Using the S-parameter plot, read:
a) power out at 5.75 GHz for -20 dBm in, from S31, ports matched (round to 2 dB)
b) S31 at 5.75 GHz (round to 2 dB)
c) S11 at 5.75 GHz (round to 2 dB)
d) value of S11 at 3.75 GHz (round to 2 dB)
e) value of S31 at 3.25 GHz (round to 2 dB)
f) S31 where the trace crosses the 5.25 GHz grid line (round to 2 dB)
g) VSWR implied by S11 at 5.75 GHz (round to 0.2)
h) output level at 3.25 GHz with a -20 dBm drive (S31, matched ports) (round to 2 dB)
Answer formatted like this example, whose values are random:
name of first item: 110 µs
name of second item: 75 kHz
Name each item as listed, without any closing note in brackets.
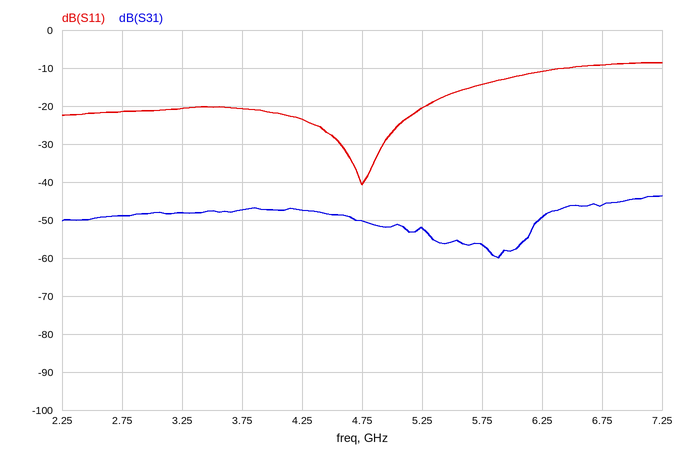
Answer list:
power out at 5.75 GHz for -20 dBm in, from S31, ports matched: -76 dBm
S31 at 5.75 GHz: -56 dB
S11 at 5.75 GHz: -14 dB
value of S11 at 3.75 GHz: -20 dB
value of S31 at 3.25 GHz: -48 dB
S31 where the trace crosses the 5.25 GHz grid line: -52 dB
VSWR implied by S11 at 5.75 GHz: 1.4
output level at 3.25 GHz with a -20 dBm drive (S31, matched ports): -68 dBm
